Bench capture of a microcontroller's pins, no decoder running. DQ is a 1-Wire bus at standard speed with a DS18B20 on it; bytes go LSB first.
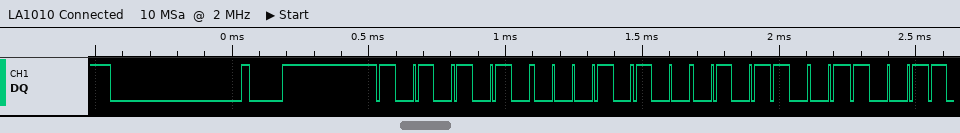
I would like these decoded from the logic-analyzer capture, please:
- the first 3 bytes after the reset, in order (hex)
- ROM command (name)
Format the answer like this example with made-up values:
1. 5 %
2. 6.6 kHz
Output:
1. 55 28 9A
2. Match ROM
